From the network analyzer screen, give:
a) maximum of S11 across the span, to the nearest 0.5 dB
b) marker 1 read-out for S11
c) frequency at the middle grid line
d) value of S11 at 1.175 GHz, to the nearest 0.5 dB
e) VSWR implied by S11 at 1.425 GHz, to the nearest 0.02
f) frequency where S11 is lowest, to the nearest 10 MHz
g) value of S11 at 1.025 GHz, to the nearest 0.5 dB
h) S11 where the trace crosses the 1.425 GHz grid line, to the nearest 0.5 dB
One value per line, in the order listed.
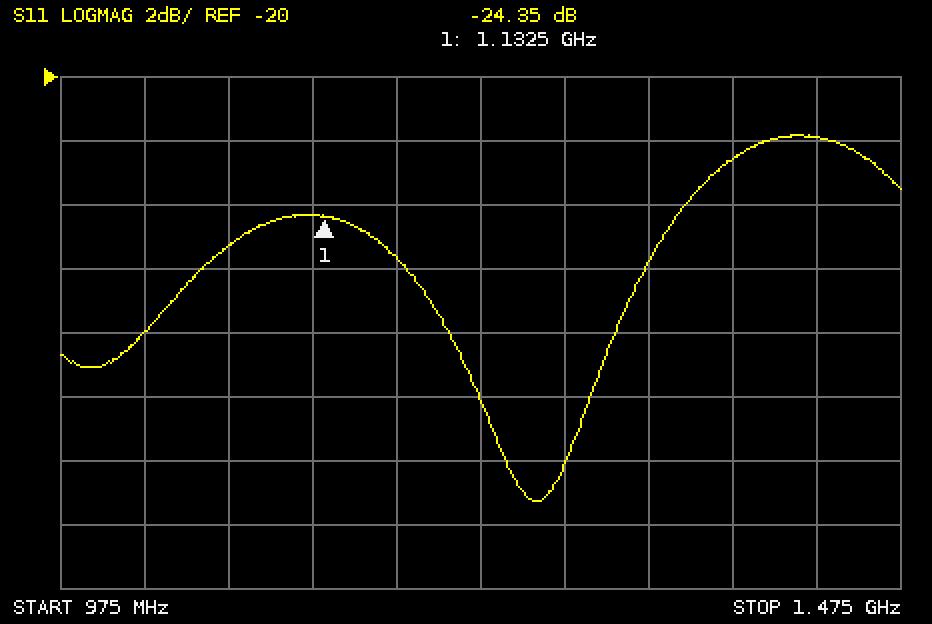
-22.0 dB
-24.35 dB
1.225 GHz
-25.5 dB
1.18
1.26 GHz
-28.0 dB
-22.0 dB
